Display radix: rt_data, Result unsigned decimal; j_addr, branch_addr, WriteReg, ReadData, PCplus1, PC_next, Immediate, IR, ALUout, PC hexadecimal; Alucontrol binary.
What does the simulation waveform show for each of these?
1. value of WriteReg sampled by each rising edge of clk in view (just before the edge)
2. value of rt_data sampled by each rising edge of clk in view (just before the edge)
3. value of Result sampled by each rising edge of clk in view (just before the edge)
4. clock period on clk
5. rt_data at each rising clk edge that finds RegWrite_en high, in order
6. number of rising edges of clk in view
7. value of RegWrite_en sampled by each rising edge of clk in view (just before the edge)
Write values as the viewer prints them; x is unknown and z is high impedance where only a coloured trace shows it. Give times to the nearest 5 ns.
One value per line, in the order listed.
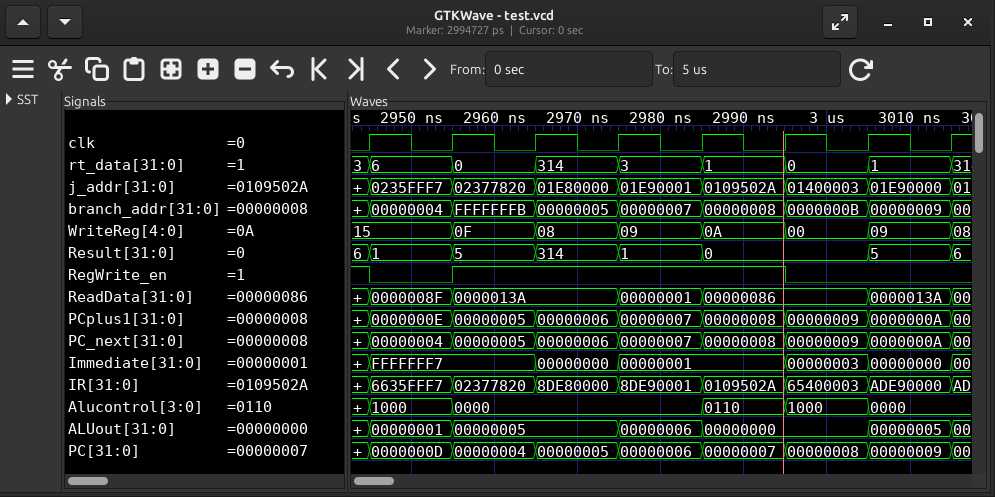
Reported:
15, 15, 0F, 08, 09, 0A, 00, 09
3, 6, 0, 314, 3, 1, 0, 1
6, 1, 5, 314, 1, 0, 0, 5
10 ns
3, 0, 314, 3, 1
8
1 0 1 1 1 1 0 0
